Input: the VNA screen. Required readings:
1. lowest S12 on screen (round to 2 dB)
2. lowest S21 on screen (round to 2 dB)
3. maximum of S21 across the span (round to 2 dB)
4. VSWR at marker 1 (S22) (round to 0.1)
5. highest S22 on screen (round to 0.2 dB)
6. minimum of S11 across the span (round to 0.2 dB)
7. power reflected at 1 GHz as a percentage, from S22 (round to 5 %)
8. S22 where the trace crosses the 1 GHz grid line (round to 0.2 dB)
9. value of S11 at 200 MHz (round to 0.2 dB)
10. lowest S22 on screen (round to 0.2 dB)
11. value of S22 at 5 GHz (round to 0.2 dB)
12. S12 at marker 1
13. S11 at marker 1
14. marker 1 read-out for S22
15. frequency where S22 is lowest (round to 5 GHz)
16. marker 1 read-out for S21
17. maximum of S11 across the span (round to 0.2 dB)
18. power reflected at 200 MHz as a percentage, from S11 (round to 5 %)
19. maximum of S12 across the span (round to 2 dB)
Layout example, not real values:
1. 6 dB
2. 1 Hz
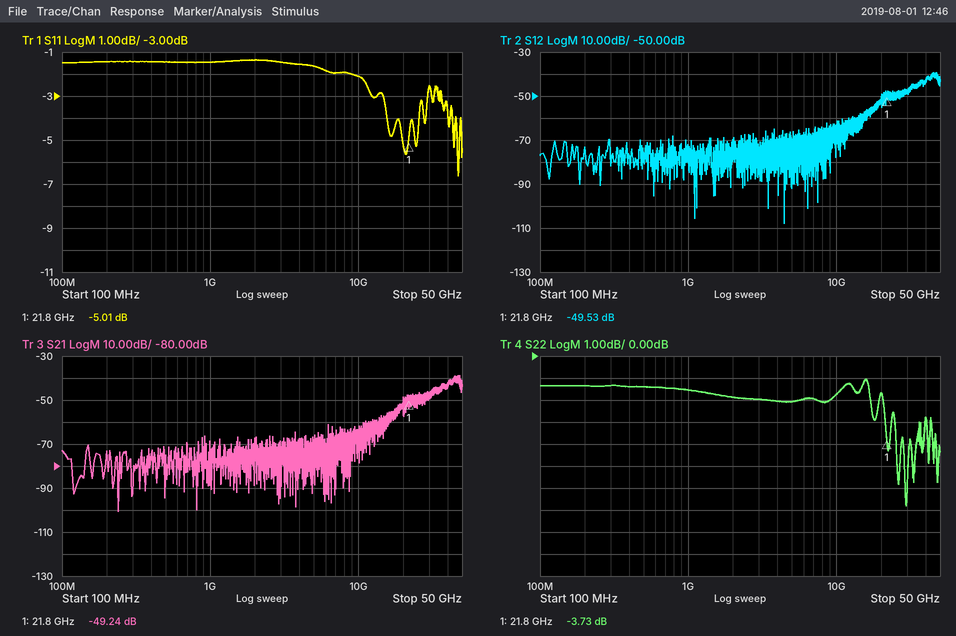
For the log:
1. -108 dB
2. -100 dB
3. -38 dB
4. 4.7
5. -1.0 dB
6. -6.6 dB
7. 70 %
8. -1.6 dB
9. -1.4 dB
10. -6.8 dB
11. -2.0 dB
12. -49.53 dB
13. -5.01 dB
14. -3.73 dB
15. 30 GHz
16. -49.24 dB
17. -1.4 dB
18. 70 %
19. -40 dB
